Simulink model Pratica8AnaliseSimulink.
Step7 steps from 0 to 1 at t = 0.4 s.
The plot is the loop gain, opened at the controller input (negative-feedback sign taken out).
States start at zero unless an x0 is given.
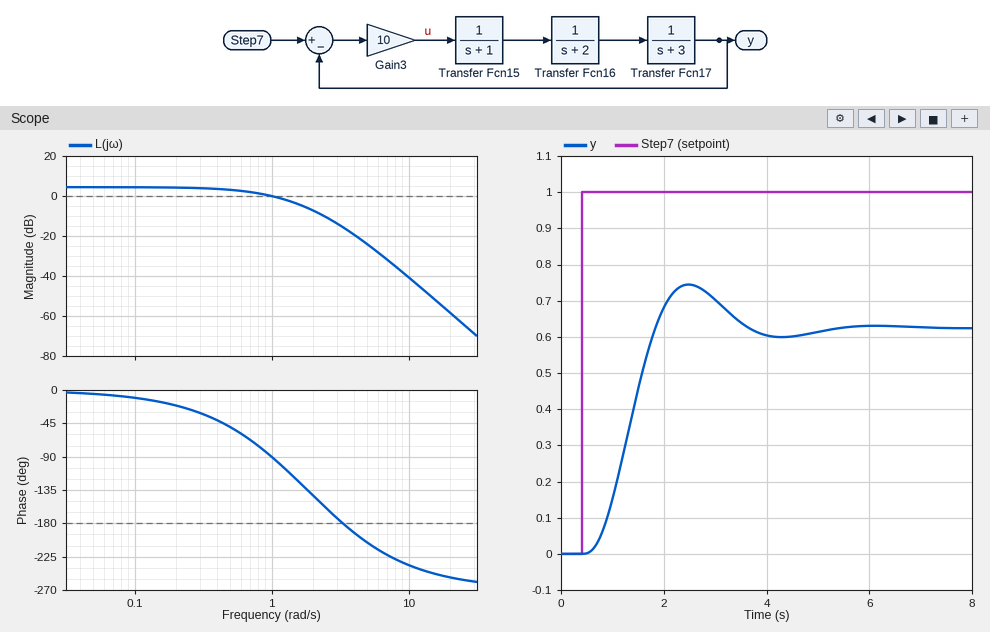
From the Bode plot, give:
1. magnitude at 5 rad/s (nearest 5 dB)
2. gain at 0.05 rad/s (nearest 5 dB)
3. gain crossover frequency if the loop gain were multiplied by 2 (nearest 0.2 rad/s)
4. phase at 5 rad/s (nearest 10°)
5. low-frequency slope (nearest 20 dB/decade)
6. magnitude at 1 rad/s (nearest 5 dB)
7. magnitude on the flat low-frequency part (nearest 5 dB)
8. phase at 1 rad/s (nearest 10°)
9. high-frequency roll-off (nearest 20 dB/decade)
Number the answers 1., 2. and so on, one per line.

1. -25 dB
2. 5 dB
3. 1.8 rad/s
4. -210°
5. 0 dB/decade
6. 0 dB
7. 5 dB
8. -90°
9. -60 dB/decade
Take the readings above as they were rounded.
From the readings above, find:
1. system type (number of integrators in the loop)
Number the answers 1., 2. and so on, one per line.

1. 0
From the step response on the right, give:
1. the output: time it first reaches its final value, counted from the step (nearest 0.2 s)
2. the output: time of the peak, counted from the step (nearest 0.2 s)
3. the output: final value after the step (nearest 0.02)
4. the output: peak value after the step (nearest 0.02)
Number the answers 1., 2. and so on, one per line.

1. 1.4 s
2. 2.0 s
3. 0.62
4. 0.74
